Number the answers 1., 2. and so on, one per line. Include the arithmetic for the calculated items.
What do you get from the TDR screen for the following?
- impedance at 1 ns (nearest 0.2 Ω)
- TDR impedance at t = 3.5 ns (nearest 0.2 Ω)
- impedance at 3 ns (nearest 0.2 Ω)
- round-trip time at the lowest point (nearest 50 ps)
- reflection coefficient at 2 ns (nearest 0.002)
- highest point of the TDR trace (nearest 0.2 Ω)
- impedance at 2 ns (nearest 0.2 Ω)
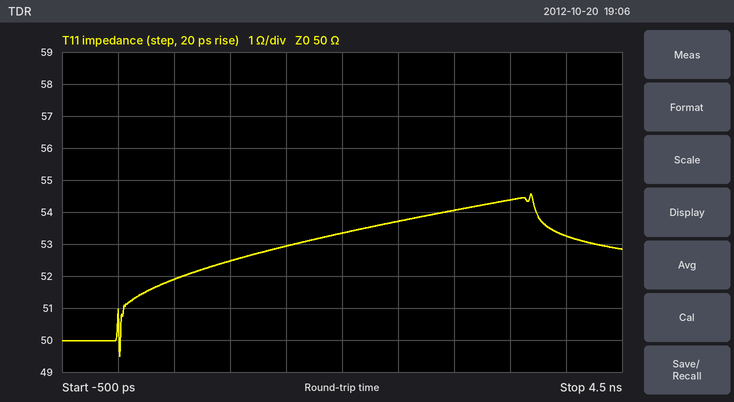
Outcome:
1. 52.4 Ω
2. 54.4 Ω
3. 54.0 Ω
4. 0 ps
5. (53.4 − 50)/(53.4 + 50) ≈ +0.0329, so +0.032 to the nearest 0.002
6. 54.6 Ω
7. 53.4 Ω
